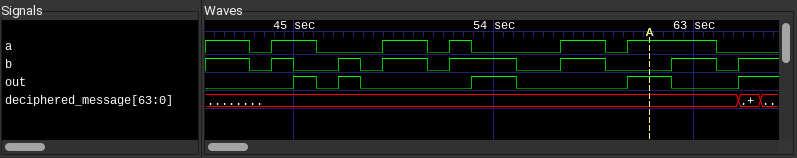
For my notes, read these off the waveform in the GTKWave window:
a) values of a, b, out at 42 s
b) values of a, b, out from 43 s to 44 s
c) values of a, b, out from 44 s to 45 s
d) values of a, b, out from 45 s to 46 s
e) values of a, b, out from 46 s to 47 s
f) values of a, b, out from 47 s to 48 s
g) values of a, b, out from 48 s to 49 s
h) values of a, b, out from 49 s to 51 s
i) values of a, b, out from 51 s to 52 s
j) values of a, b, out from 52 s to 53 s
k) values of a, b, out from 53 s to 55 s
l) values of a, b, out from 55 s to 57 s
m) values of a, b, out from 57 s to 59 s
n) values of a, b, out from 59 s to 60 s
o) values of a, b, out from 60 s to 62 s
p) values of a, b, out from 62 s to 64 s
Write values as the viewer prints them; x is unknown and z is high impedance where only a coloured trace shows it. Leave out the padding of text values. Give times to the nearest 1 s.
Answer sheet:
a=1, b=1, out=0
a=0, b=0, out=0
a=1, b=1, out=0
a=1, b=0, out=1
a=0, b=0, out=0
a=0, b=1, out=1
a=0, b=0, out=0
a=1, b=1, out=0
a=0, b=0, out=0
a=1, b=1, out=0
a=0, b=1, out=1
a=0, b=0, out=0
a=1, b=1, out=0
a=0, b=0, out=0
a=1, b=0, out=1
a=1, b=1, out=0
